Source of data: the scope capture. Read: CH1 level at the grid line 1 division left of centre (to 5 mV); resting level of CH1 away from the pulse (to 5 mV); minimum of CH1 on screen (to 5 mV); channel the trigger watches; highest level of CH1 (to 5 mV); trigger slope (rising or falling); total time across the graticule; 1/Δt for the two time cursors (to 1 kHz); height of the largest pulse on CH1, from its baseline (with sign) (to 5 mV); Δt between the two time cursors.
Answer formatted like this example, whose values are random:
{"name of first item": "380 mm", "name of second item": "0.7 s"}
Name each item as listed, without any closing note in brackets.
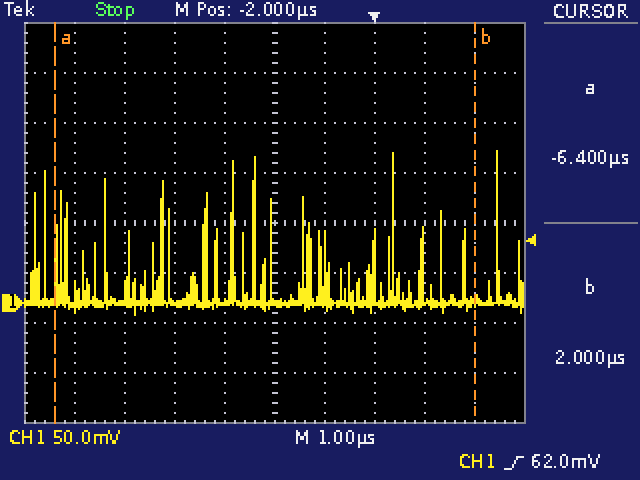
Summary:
{"CH1 level at the grid line 1 division left of centre": "0 mV", "resting level of CH1 away from the pulse": "0 mV", "minimum of CH1 on screen": "-10 mV", "channel the trigger watches": "CH1", "highest level of CH1": "150 mV", "trigger slope": "rising", "total time across the graticule": "10 µs", "1/Δt for the two time cursors": "119 kHz", "height of the largest pulse on CH1, from its baseline (with sign)": "+150 mV", "Δt between the two time cursors": "8.4 µs"}
